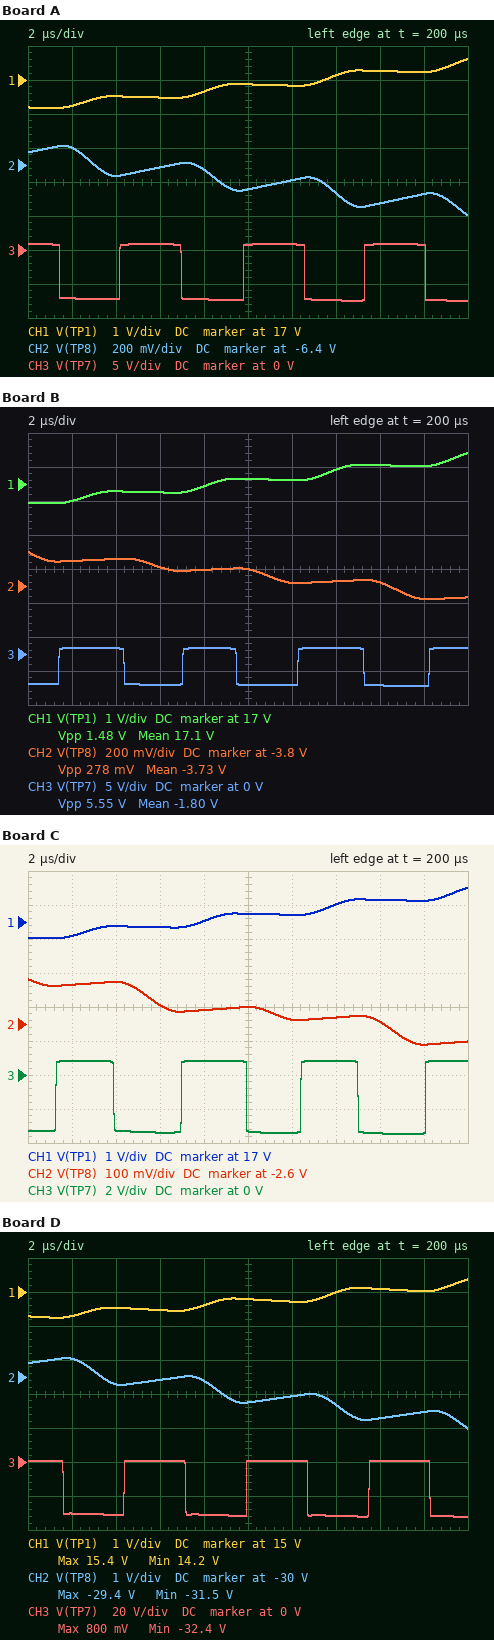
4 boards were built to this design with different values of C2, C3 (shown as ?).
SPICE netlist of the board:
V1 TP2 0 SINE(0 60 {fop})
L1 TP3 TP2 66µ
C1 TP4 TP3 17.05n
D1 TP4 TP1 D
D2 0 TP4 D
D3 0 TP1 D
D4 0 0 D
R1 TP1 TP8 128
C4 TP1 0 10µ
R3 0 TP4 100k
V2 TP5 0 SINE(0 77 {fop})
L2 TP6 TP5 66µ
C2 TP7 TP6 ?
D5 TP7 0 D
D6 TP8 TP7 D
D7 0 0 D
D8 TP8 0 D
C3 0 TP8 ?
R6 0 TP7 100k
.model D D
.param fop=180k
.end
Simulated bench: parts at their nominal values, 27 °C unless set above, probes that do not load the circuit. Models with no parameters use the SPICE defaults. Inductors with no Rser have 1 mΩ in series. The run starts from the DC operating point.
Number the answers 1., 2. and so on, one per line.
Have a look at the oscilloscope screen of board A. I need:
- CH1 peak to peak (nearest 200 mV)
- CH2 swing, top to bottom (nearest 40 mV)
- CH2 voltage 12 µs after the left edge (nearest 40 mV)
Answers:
1. 1.4 V
2. 400 mV
3. -6.48 V
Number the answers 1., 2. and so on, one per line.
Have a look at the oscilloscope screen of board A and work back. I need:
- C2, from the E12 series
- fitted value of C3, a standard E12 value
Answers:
1. 5.6 nF
2. 6.8 µF
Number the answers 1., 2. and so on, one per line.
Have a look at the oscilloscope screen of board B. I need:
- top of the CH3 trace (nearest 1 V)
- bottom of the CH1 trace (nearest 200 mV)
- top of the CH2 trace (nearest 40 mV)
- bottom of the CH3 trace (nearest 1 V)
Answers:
1. 1 V
2. 16.4 V
3. -3.60 V
4. -5 V
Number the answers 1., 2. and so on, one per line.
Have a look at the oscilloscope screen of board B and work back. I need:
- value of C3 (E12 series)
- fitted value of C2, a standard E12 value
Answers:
1. 27 µF
2. 33 nF
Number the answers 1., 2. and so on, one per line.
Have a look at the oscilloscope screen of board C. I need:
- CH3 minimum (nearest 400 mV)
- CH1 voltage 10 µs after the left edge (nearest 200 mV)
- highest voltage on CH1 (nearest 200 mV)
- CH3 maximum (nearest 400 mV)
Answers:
1. -3.6 V
2. 17.2 V
3. 18.0 V
4. 800 mV
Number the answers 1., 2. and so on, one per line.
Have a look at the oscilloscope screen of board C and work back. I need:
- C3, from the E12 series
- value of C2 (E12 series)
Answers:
1. 33 µF
2. 47 nF
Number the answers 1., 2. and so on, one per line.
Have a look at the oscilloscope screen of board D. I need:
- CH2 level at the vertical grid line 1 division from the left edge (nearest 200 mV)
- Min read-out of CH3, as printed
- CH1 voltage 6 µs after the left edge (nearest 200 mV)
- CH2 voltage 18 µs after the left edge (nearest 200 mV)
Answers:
1. -29.4 V
2. -32.4 V
3. 14.4 V
4. -31.0 V
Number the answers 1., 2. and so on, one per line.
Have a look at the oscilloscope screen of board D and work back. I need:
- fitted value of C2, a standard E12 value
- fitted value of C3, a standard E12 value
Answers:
1. 8.2 nF
2. 3.9 µF
